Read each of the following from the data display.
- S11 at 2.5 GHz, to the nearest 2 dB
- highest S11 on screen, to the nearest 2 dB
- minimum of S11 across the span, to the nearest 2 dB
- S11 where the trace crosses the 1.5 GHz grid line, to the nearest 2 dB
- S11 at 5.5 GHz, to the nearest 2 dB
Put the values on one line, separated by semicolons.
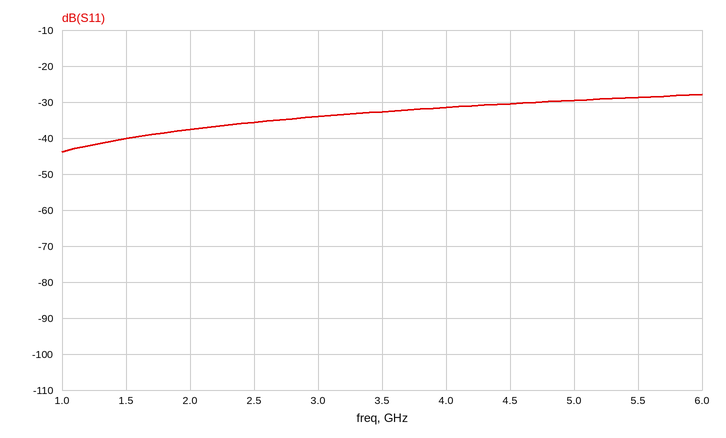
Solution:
-36 dB; -28 dB; -44 dB; -40 dB; -28 dB
